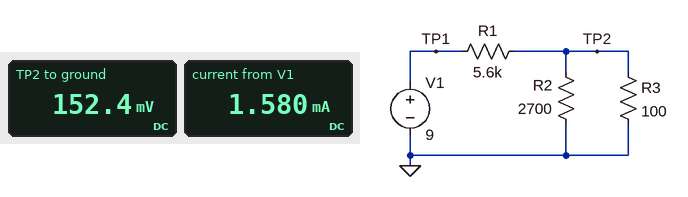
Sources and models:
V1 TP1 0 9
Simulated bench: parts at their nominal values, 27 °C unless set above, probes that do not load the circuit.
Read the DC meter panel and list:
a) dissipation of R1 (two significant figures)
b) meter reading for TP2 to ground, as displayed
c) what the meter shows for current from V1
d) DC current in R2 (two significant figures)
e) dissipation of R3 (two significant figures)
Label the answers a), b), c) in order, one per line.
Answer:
a) 14 mW
b) 152.4 mV
c) 1.580 mA
d) 56 µA
e) 230 µW
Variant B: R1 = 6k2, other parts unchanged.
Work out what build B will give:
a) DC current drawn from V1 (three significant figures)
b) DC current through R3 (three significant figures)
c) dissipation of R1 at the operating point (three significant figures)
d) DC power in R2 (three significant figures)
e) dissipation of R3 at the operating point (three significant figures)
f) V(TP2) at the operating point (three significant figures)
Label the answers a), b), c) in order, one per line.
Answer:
a) 1.43 mA
b) 1.38 mA
c) 12.7 mW
d) 7.04 µW
e) 190 µW
f) 138 mV
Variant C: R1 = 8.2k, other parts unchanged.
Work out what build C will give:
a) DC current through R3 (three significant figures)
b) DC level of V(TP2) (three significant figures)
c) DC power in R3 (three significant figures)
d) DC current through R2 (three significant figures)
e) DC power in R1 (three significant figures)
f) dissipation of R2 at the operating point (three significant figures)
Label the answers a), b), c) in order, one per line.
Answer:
a) 1.05 mA
b) 105 mV
c) 109 µW
d) 38.7 µA
e) 9.65 mW
f) 4.05 µW
